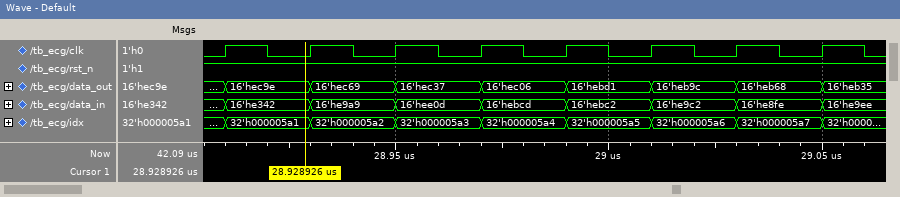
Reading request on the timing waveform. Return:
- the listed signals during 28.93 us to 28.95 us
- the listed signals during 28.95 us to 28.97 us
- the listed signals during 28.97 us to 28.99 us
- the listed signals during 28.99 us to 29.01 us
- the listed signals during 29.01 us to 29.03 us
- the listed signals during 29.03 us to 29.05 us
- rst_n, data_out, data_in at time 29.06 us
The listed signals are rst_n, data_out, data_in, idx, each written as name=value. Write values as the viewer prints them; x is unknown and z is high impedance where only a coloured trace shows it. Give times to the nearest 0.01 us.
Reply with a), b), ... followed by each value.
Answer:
a) rst_n=1, data_out=16'hec69, data_in=16'he9a9, idx=32'h000005a2
b) rst_n=1, data_out=16'hec37, data_in=16'hee0d, idx=32'h000005a3
c) rst_n=1, data_out=16'hec06, data_in=16'hebcd, idx=32'h000005a4
d) rst_n=1, data_out=16'hebd1, data_in=16'hebc2, idx=32'h000005a5
e) rst_n=1, data_out=16'heb9c, data_in=16'he9c2, idx=32'h000005a6
f) rst_n=1, data_out=16'heb68, data_in=16'he8fe, idx=32'h000005a7
g) rst_n=1, data_out=16'heb35, data_in=16'he9ee
